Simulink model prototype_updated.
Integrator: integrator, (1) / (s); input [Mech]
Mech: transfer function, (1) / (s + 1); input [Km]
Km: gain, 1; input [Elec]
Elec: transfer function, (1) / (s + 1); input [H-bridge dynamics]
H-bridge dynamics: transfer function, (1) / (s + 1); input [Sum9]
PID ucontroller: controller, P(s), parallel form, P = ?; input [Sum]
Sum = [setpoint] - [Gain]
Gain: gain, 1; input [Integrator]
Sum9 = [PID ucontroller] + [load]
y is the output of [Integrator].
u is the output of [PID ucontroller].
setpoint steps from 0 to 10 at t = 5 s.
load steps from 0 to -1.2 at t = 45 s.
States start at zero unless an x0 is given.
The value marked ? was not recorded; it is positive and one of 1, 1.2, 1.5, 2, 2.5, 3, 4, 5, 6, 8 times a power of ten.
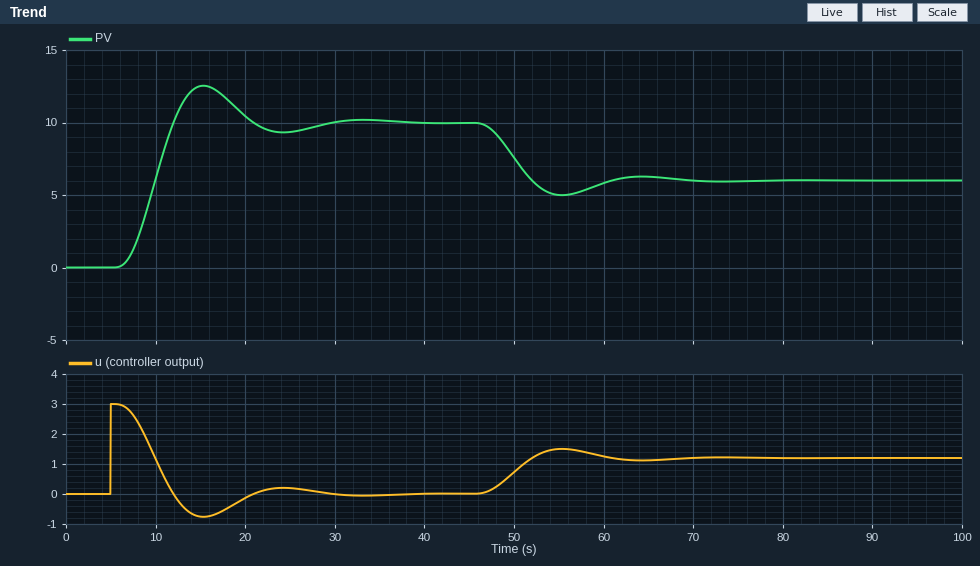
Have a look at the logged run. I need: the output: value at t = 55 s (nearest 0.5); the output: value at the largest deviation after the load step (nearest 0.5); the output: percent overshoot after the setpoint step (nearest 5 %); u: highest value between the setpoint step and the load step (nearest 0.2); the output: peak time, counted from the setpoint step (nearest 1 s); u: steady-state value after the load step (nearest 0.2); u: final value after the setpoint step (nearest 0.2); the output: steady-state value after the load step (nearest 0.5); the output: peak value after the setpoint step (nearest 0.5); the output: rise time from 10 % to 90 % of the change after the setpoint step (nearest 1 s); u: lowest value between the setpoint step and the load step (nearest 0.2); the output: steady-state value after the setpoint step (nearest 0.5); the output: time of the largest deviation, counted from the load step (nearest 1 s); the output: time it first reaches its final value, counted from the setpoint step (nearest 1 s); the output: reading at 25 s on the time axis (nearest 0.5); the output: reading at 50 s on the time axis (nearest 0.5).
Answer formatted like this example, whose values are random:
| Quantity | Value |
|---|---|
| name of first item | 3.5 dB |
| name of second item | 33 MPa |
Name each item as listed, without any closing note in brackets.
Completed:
| Quantity | Value |
|---|---|
| the output: value at t = 55 s | 5.0 |
| the output: value at the largest deviation after the load step | 5.0 |
| the output: percent overshoot after the setpoint step | 25 % |
| u: highest value between the setpoint step and the load step | 3.0 |
| the output: peak time, counted from the setpoint step | 10 s |
| u: steady-state value after the load step | 1.2 |
| u: final value after the setpoint step | 0.0 |
| the output: steady-state value after the load step | 6.0 |
| the output: peak value after the setpoint step | 12.5 |
| the output: rise time from 10 % to 90 % of the change after the setpoint step | 4 s |
| u: lowest value between the setpoint step and the load step | -0.8 |
| the output: steady-state value after the setpoint step | 10.0 |
| the output: time of the largest deviation, counted from the load step | 10 s |
| the output: time it first reaches its final value, counted from the setpoint step | 7 s |
| the output: reading at 25 s on the time axis | 9.5 |
| the output: reading at 50 s on the time axis | 7.5 |
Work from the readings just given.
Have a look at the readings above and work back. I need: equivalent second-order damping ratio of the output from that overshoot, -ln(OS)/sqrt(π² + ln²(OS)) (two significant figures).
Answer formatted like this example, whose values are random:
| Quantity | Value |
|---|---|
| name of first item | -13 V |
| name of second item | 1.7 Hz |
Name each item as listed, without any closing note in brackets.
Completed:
| Quantity | Value |
|---|---|
| equivalent second-order damping ratio of the output from that overshoot, -ln(OS)/sqrt(π² + ln²(OS)) | 0.40 |
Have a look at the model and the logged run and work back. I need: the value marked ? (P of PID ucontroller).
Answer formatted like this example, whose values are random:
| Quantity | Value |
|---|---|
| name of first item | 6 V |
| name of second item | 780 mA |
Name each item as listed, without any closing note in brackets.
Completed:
| Quantity | Value |
|---|---|
| the value marked ? | 0.3 |
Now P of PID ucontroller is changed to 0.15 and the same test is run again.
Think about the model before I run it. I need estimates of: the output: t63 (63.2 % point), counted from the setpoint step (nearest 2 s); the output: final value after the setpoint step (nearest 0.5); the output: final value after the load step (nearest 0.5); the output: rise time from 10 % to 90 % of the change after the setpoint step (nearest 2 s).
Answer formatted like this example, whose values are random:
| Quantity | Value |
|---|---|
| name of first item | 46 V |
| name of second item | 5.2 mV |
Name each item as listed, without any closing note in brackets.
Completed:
| Quantity | Value |
|---|---|
| the output: t63 (63.2 % point), counted from the setpoint step | 8 s |
| the output: final value after the setpoint step | 10.0 |
| the output: final value after the load step | 2.0 |
| the output: rise time from 10 % to 90 % of the change after the setpoint step | 8 s |
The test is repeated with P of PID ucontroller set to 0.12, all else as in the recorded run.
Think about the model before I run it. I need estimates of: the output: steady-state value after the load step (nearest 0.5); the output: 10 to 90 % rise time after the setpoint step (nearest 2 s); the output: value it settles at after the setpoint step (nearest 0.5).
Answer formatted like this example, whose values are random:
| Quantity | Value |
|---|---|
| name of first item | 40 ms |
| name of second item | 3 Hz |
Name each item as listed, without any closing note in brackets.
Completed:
| Quantity | Value |
|---|---|
| the output: steady-state value after the load step | 0.0 |
| the output: 10 to 90 % rise time after the setpoint step | 12 s |
| the output: value it settles at after the setpoint step | 10.0 |
